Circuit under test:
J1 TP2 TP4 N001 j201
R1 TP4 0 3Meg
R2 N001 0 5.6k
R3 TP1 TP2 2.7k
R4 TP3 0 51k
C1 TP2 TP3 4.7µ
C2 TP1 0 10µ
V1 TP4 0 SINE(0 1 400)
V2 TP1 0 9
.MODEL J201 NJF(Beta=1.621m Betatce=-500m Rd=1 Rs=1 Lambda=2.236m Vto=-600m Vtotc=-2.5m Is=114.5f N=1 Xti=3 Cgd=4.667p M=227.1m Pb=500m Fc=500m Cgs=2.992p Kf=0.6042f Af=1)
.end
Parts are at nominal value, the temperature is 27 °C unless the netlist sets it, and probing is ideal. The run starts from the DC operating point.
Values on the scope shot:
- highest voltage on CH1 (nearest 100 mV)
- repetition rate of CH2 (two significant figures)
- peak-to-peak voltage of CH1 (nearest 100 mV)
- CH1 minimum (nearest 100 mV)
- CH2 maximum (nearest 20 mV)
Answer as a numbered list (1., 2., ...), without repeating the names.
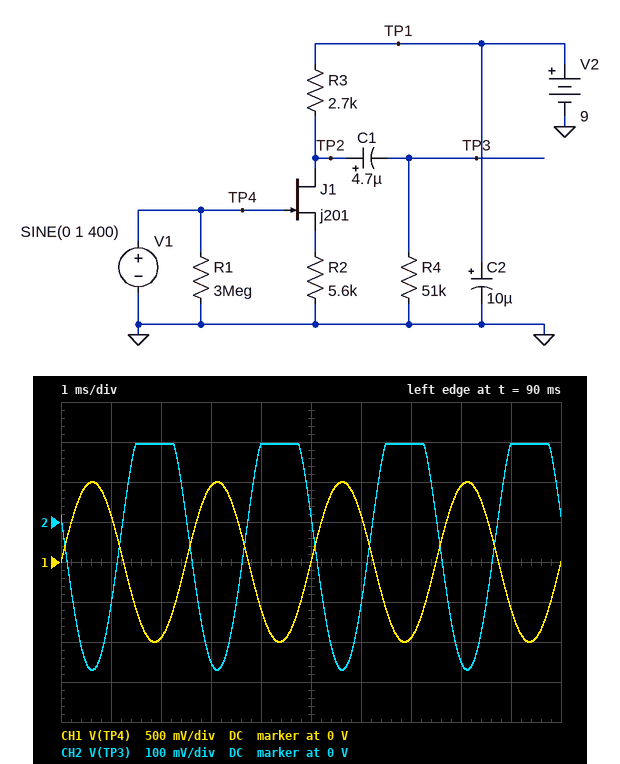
1. 1.0 V
2. 400 Hz
3. 2.0 V
4. -1.0 V
5. 200 mV
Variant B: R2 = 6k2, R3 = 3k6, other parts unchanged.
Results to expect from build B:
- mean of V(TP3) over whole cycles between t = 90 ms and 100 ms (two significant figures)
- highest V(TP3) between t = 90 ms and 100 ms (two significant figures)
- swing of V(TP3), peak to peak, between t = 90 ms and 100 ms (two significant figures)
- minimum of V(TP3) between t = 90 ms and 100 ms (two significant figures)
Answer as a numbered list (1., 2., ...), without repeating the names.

1. -38 mV
2. 240 mV
3. 680 mV
4. -440 mV
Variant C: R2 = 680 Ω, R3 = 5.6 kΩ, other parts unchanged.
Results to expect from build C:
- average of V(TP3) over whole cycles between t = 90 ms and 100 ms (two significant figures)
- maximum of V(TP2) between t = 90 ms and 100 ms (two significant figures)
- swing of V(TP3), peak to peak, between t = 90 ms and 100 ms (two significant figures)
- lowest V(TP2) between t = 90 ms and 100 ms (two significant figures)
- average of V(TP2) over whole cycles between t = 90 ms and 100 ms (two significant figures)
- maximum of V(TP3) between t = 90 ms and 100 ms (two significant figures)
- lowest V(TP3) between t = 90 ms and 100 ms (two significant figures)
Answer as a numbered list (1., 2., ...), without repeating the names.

1. -510 mV
2. 8.8 V
3. 5.7 V
4. 3.1 V
5. 6.7 V
6. 1.6 V
7. -4.1 V
